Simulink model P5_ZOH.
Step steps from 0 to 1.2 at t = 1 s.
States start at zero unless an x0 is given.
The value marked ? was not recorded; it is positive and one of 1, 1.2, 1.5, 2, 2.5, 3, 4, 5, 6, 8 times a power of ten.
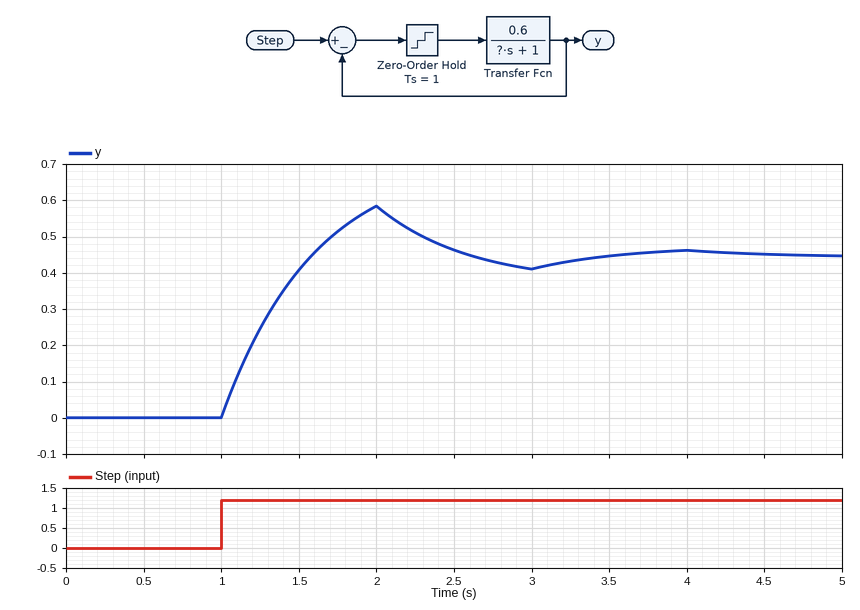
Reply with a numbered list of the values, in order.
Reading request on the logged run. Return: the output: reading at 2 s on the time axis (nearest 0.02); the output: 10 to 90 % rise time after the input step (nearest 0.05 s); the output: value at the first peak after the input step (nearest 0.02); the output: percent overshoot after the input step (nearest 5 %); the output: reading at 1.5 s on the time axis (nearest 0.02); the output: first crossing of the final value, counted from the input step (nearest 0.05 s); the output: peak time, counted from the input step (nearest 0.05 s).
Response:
1. 0.58
2. 0.45 s
3. 0.58
4. 30 %
5. 0.40
6. 0.60 s
7. 1.00 s
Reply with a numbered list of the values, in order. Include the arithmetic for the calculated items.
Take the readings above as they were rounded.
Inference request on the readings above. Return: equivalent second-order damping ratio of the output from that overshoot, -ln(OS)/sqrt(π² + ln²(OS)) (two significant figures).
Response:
1. ln(0.3) = -1.204; 1.204 / sqrt(9.870 + 1.450) = 0.36
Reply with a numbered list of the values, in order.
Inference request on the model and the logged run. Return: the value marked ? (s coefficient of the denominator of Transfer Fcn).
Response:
1. 0.6
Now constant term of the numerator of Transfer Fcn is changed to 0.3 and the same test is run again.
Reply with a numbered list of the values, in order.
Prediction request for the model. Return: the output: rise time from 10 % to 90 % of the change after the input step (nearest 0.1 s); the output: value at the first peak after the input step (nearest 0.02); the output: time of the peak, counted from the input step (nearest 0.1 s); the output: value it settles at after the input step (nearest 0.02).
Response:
1. 0.7 s
2. 0.30
3. 1.0 s
4. 0.28
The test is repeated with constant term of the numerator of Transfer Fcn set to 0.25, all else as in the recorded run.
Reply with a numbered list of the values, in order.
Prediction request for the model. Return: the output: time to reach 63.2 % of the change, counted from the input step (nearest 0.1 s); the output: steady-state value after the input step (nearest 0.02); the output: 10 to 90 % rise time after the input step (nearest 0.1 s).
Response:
1. 0.4 s
2. 0.24
3. 0.7 s
